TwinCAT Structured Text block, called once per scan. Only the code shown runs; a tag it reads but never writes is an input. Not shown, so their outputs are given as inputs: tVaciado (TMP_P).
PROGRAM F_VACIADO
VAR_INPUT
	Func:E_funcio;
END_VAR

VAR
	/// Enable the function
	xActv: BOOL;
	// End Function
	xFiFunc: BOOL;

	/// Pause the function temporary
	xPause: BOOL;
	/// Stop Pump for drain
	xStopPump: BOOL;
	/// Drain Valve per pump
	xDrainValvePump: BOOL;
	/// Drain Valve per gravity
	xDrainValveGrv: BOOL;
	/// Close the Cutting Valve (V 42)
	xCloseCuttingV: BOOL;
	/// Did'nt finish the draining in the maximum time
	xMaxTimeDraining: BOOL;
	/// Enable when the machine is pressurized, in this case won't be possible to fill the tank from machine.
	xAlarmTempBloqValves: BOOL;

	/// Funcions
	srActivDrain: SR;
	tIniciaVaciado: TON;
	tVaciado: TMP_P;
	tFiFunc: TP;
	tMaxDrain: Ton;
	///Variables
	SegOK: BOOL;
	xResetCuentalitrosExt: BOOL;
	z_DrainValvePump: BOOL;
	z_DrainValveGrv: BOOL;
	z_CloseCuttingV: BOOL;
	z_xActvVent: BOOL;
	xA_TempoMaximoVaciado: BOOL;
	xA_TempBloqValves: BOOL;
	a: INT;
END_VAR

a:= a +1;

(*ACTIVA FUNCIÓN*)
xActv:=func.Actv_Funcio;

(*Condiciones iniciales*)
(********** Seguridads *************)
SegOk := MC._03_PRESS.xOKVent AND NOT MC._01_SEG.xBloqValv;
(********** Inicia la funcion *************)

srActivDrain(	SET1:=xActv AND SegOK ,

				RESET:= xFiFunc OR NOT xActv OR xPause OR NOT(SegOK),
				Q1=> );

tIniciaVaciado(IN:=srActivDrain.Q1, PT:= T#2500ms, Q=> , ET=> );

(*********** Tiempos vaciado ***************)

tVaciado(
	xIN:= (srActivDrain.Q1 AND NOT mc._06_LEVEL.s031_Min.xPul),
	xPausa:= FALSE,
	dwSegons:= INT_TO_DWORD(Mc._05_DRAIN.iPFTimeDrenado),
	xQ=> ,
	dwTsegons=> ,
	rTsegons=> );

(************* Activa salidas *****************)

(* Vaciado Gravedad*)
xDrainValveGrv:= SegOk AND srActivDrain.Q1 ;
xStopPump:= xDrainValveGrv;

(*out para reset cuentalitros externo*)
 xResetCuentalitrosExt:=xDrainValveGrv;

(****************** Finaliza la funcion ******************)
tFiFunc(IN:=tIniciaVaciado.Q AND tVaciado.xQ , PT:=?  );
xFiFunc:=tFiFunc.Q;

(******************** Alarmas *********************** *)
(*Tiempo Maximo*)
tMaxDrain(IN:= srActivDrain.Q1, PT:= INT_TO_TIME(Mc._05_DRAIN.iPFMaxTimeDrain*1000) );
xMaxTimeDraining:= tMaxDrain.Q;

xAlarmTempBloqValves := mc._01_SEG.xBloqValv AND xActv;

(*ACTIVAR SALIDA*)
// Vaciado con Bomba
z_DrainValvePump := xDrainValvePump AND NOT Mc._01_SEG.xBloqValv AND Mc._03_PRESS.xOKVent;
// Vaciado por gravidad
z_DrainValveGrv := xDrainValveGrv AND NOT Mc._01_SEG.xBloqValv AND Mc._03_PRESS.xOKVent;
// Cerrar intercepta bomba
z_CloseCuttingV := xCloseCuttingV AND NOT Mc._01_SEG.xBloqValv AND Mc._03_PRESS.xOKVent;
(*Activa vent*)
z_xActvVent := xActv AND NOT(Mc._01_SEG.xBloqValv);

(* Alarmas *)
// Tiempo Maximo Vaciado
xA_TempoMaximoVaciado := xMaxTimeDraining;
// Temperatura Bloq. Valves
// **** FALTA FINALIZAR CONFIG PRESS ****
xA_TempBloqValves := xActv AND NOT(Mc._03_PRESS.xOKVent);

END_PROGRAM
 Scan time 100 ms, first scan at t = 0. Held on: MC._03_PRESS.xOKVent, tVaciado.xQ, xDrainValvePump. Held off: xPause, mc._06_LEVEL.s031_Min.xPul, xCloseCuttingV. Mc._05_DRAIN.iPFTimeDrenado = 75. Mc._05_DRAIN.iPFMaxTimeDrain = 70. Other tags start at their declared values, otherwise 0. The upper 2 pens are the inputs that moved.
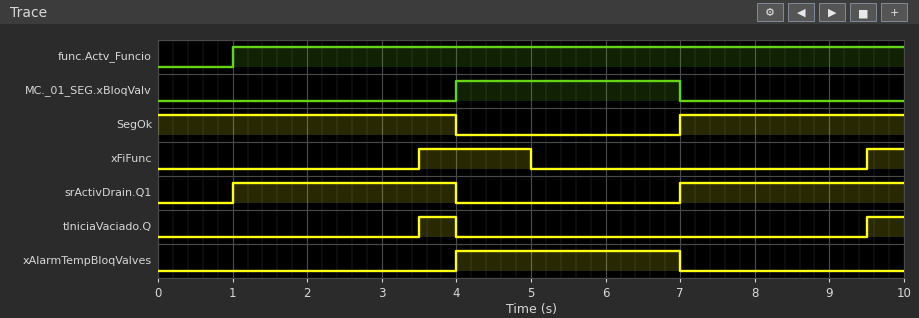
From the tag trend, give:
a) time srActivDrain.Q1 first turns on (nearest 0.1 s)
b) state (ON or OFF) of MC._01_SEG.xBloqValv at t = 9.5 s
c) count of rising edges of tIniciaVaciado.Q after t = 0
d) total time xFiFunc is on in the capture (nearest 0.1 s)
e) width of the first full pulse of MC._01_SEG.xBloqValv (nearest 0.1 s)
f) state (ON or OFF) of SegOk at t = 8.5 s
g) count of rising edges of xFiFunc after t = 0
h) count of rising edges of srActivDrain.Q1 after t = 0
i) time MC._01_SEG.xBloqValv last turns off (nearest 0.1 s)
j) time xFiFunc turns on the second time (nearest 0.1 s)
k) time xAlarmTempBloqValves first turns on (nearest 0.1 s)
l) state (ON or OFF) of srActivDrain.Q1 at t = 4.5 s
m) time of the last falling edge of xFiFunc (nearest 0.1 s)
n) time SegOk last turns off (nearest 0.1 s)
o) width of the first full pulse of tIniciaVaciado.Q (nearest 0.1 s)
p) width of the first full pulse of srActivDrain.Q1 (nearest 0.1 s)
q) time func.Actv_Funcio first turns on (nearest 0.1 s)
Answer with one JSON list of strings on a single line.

["1.0 s", "OFF", "2", "2.0 s", "3.0 s", "ON", "2", "2", "7.0 s", "9.5 s", "4.0 s", "OFF", "5.0 s", "4.0 s", "0.5 s", "3.0 s", "1.0 s"]
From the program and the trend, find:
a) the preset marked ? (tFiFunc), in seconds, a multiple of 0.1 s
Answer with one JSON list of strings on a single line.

["1.5 s"]
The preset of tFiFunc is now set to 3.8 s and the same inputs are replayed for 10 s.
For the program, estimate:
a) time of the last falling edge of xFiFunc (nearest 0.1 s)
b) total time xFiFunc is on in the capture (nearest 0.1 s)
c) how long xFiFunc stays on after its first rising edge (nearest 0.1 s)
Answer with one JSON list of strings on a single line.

["7.3 s", "4.3 s", "3.8 s"]
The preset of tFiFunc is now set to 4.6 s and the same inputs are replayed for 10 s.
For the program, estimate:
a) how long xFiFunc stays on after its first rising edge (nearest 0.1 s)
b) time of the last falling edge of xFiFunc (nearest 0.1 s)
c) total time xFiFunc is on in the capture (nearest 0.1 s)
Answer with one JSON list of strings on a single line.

["4.6 s", "8.1 s", "5.1 s"]
